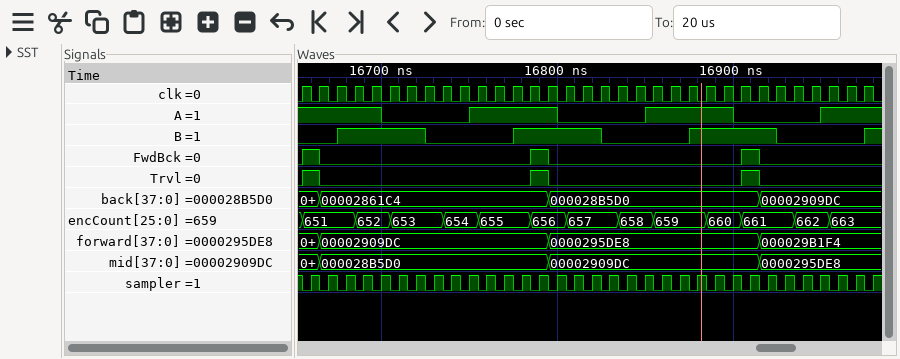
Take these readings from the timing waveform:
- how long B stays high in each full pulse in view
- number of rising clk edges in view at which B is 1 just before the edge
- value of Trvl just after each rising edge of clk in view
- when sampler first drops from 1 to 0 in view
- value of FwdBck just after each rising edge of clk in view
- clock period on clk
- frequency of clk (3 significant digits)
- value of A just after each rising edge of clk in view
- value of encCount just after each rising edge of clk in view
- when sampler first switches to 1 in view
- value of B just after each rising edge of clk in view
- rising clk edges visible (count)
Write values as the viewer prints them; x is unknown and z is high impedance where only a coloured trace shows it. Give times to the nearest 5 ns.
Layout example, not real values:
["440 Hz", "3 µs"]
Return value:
["50 ns, 50 ns, 50 ns", "15", "1 0 0 0 0 0 0 0 0 0 0 0 0 1 0 0 0 0 0 0 0 0 0 0 0 1 0 0 0 0 0 0 0", "16655 ns", "1 0 0 0 0 0 0 0 0 0 0 0 0 1 0 0 0 0 0 0 0 0 0 0 0 1 0 0 0 0 0 0 0", "10 ns", "100 MHz", "1 1 1 1 1 0 0 0 0 0 1 1 1 1 1 0 0 0 0 0 1 1 1 1 1 0 0 0 0 0 1 1 1", "651, 651, 651, 652, 652, 653, 653, 653, 654, 654, 655, 655, 655, 656, 656, 657, 657, 657, 658, 658, 659, 659, 659, 660, 660, 661, 661, 661, 662, 662, 663, 663, 663", "16660 ns", "0 0 1 1 1 1 1 0 0 0 0 0 1 1 1 1 1 0 0 0 0 0 1 1 1 1 1 0 0 0 0 0 1", "33"]
